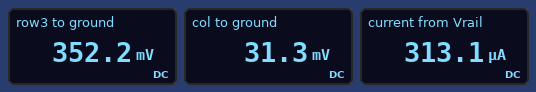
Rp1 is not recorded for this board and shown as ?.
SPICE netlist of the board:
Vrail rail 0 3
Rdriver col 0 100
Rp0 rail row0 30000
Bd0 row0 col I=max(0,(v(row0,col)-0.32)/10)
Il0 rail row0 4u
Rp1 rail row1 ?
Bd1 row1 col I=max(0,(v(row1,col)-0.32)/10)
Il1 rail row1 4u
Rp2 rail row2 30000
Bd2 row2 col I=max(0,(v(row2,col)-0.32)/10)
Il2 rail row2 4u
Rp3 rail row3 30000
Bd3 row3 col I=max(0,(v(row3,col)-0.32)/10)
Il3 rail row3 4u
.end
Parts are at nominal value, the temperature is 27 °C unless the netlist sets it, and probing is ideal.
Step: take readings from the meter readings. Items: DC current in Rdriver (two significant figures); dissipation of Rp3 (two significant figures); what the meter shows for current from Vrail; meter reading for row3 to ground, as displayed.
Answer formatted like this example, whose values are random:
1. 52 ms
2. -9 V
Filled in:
1. 310 µA
2. 230 µW
3. 313.1 µA
4. 352.2 mV
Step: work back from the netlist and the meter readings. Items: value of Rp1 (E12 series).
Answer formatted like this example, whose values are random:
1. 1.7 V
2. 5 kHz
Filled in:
1. 82 kΩ
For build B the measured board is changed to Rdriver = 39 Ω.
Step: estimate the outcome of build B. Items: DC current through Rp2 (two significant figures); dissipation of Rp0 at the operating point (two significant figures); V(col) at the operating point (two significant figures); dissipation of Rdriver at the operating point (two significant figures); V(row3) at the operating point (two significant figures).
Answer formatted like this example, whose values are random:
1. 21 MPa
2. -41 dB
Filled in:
1. 89 µA
2. 240 µW
3. 12 mV
4. 3.9 µW
5. 330 mV
